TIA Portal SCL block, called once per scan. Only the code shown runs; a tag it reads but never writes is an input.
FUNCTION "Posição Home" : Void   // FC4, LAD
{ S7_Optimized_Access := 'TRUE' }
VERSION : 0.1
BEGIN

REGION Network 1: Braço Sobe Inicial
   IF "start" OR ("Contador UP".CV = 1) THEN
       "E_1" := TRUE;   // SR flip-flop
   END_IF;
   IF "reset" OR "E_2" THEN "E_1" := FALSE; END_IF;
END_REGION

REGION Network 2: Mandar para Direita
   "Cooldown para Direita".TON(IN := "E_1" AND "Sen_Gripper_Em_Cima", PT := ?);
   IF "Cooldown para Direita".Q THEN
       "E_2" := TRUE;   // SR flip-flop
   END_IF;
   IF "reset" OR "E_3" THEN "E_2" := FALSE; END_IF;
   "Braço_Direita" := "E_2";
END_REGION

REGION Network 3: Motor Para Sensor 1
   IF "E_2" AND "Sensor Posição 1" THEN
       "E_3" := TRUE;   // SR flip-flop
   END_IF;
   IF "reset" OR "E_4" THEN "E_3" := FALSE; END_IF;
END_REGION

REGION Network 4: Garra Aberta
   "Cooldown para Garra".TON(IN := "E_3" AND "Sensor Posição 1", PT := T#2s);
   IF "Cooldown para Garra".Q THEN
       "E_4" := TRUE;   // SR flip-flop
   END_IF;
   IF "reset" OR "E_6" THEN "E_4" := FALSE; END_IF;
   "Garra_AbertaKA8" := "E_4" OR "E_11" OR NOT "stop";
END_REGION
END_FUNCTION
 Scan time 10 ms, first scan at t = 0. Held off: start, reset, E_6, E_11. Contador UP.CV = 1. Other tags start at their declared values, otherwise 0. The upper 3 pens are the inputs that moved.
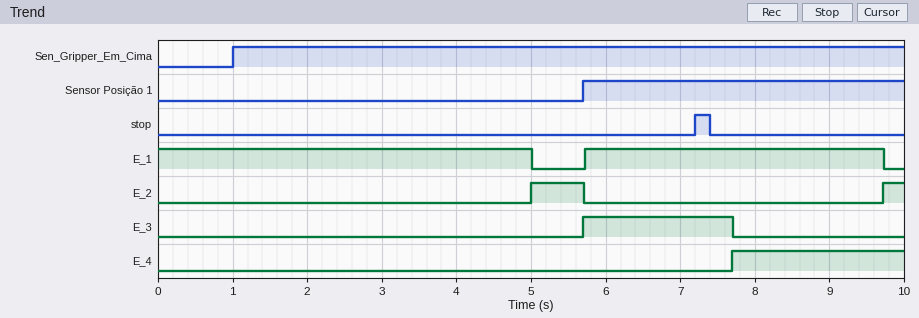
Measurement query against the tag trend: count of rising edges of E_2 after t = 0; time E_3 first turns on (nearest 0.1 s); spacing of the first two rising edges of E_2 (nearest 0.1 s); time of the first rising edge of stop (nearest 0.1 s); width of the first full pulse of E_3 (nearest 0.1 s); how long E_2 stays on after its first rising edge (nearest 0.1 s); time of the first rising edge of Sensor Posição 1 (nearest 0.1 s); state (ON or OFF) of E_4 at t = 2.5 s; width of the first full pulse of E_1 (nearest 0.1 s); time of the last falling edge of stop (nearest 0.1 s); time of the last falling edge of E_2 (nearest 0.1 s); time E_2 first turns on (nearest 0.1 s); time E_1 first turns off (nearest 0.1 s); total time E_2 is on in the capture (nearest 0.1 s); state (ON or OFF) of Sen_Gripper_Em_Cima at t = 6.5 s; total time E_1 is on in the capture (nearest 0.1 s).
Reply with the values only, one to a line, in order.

2
5.7 s
4.7 s
7.2 s
2.0 s
0.7 s
5.7 s
OFF
4.0 s
7.4 s
5.7 s
5.0 s
5.0 s
1.0 s
ON
9.0 s
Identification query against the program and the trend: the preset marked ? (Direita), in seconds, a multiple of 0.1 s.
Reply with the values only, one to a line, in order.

4.0 s
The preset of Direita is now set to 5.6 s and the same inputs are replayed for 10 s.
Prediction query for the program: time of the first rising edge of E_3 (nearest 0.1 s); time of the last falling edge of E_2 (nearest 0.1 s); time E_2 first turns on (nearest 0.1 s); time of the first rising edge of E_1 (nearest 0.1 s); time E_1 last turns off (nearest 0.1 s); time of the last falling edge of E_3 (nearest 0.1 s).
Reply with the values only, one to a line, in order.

6.6 s
6.6 s
6.6 s
6.6 s
6.6 s
8.6 s
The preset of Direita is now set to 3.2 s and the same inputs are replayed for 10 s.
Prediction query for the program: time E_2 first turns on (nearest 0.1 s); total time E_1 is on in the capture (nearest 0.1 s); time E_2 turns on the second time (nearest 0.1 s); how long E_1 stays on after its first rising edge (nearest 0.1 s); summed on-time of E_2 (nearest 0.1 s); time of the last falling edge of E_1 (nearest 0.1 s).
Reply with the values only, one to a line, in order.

4.2 s
7.4 s
8.9 s
3.2 s
2.6 s
8.9 s
